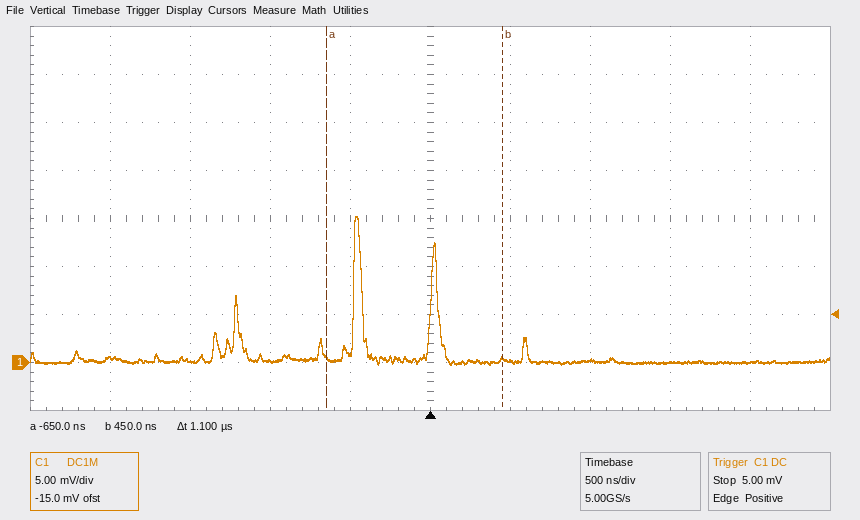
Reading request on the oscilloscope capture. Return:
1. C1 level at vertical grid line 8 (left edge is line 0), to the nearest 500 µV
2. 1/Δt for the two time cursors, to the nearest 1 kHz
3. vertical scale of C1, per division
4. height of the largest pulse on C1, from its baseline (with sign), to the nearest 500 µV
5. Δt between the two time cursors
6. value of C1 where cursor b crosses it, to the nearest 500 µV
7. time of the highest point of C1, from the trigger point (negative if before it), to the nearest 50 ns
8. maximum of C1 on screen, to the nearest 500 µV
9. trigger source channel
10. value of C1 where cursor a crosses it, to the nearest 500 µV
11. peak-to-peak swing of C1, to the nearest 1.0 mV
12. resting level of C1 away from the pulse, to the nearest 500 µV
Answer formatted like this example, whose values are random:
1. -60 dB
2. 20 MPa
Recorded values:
1. 0.0 mV
2. 909 kHz
3. 5 mV
4. +15.0 mV
5. 1.1 µs
6. 500 µV
7. -450 ns
8. 15.0 mV
9. C1
10. 500 µV
11. 15.0 mV
12. 0.0 mV
